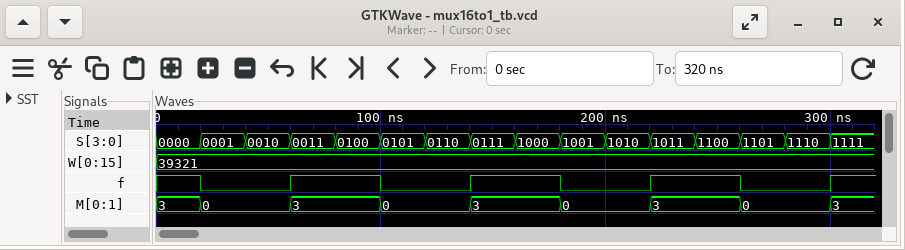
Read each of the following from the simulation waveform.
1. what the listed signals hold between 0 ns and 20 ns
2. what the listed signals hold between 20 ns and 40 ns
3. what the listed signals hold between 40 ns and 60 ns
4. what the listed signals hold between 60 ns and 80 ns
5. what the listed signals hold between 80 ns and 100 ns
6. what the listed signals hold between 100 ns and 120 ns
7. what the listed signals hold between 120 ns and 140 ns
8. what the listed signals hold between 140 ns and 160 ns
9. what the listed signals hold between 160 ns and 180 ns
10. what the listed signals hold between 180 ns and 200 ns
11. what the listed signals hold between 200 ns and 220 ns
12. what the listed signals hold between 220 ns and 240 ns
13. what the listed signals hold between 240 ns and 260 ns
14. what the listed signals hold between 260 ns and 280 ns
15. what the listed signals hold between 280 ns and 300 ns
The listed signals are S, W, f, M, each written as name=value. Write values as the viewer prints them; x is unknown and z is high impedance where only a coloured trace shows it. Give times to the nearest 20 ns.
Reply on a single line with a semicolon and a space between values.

S=0000, W=39321, f=1, M=3; S=0001, W=39321, f=0, M=0; S=0010, W=39321, f=0, M=0; S=0011, W=39321, f=1, M=3; S=0100, W=39321, f=1, M=3; S=0101, W=39321, f=0, M=0; S=0110, W=39321, f=0, M=0; S=0111, W=39321, f=1, M=3; S=1000, W=39321, f=1, M=3; S=1001, W=39321, f=0, M=0; S=1010, W=39321, f=0, M=0; S=1011, W=39321, f=1, M=3; S=1100, W=39321, f=1, M=3; S=1101, W=39321, f=0, M=0; S=1110, W=39321, f=0, M=0
